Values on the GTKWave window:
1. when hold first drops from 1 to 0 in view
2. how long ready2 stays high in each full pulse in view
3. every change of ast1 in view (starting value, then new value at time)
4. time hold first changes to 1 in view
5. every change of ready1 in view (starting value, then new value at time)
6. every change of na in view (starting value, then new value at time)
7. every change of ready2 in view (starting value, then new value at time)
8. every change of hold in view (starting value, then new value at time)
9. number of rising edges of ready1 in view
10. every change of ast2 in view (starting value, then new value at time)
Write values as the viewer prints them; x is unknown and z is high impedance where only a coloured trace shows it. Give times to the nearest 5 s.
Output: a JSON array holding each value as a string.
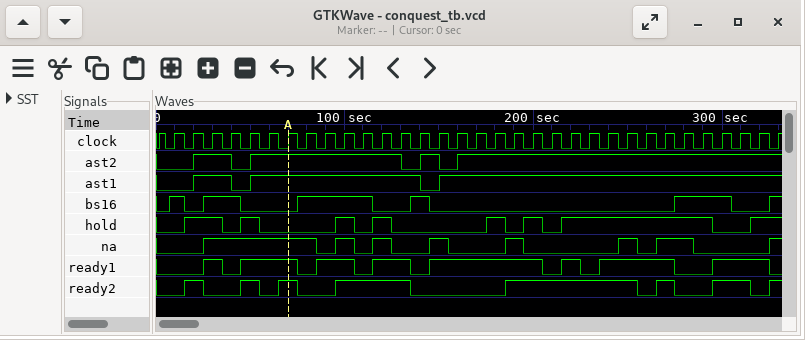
["35 s", "10 s, 10 s, 10 s, 40 s, 70 s, 10 s, 20 s", "0, 1 at 20 s, 0 at 40 s, 1 at 50 s, 0 at 140 s, 1 at 150 s", "15 s", "0, 1 at 25 s, 0 at 35 s, 1 at 45 s, 0 at 75 s, 1 at 85 s, 0 at 105 s, 1 at 115 s, 0 at 135 s, 1 at 145 s, 0 at 205 s, 1 at 215 s, 0 at 225 s, 1 at 235 s, 0 at 275 s, 1 at 295 s, 0 at 325 s", "0, 1 at 25 s, 0 at 85 s, 1 at 95 s, 0 at 105 s, 1 at 115 s, 0 at 125 s, 1 at 145 s, 0 at 155 s, 1 at 185 s, 0 at 195 s, 1 at 245 s, 0 at 255 s, 1 at 265 s, 0 at 285 s, 1 at 325 s", "0, 1 at 15 s, 0 at 25 s, 1 at 45 s, 0 at 55 s, 1 at 65 s, 0 at 75 s, 1 at 95 s, 0 at 135 s, 1 at 185 s, 0 at 255 s, 1 at 265 s, 0 at 275 s, 1 at 295 s, 0 at 315 s, 1 at 325 s", "0, 1 at 15 s, 0 at 35 s, 1 at 45 s, 0 at 55 s, 1 at 95 s, 0 at 105 s, 1 at 115 s, 0 at 125 s, 1 at 175 s, 0 at 185 s, 1 at 195 s, 0 at 205 s, 1 at 215 s, 0 at 295 s, 1 at 315 s", "8", "0, 1 at 20 s, 0 at 40 s, 1 at 50 s, 0 at 130 s, 1 at 140 s, 0 at 150 s, 1 at 160 s"]
